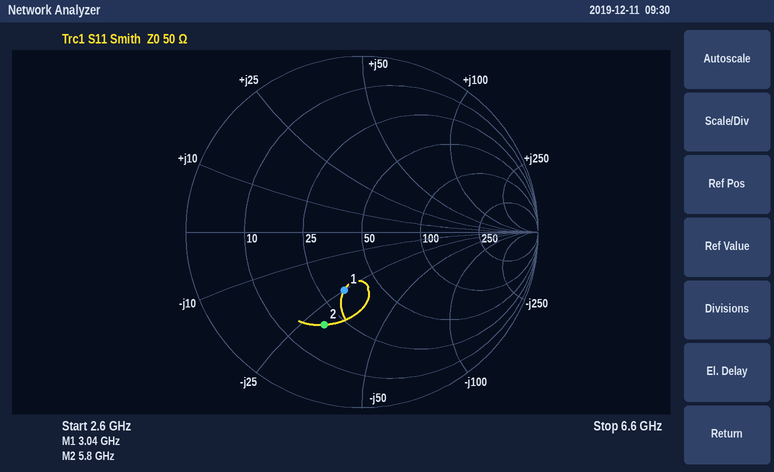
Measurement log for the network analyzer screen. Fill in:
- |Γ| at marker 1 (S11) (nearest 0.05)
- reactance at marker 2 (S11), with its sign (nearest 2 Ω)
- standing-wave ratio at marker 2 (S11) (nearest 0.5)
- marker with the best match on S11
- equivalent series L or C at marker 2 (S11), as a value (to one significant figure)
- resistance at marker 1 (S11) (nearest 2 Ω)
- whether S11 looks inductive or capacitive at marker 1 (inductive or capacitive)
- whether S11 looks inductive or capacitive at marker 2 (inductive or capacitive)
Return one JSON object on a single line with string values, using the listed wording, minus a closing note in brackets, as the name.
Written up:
{"|Γ| at marker 1 (S11)": "0.35", "reactance at marker 2 (S11), with its sign": "-30 Ω", "standing-wave ratio at marker 2 (S11)": "3.5", "marker with the best match on S11": "marker 1", "equivalent series L or C at marker 2 (S11), as a value": "900 fF", "resistance at marker 1 (S11)": "34 Ω", "whether S11 looks inductive or capacitive at marker 1": "capacitive", "whether S11 looks inductive or capacitive at marker 2": "capacitive"}
